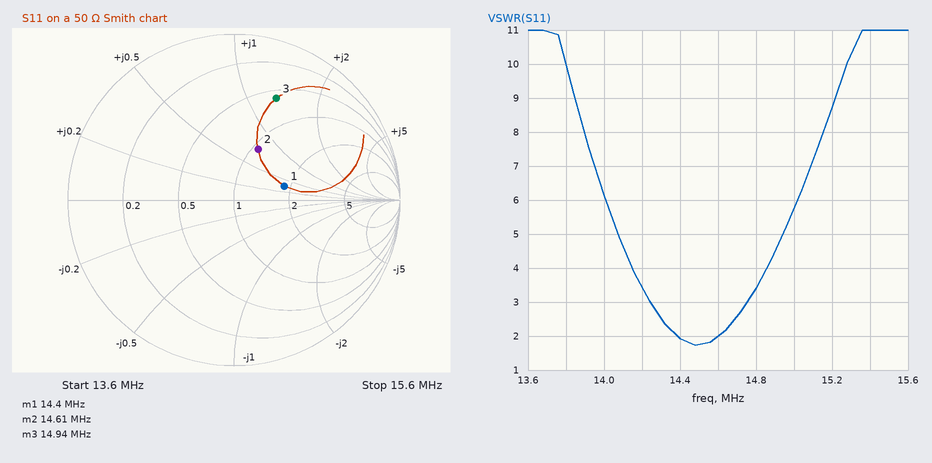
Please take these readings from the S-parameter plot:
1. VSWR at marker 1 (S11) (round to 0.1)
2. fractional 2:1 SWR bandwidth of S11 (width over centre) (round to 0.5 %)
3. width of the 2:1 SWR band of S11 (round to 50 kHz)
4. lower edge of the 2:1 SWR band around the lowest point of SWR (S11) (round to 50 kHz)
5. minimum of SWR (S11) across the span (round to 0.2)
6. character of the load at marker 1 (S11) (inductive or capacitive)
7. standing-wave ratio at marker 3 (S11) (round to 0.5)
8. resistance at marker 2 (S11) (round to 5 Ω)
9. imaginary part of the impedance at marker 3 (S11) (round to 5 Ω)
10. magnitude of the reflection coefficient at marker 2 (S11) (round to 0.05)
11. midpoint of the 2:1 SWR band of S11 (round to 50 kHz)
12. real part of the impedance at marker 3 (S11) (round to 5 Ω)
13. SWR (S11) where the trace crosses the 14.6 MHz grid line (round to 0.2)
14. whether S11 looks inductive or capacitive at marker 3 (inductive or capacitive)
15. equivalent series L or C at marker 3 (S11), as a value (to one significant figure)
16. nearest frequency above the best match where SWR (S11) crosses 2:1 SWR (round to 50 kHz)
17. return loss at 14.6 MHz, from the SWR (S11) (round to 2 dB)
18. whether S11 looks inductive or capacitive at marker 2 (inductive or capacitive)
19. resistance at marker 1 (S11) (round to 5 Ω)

1.9
1.5 %
200 kHz
14.40 MHz
1.8
inductive
5.0
55 Ω
+65 Ω
0.35
14.50 MHz
30 Ω
2.0
inductive
700 nH
14.60 MHz
10 dB
inductive
90 Ω
